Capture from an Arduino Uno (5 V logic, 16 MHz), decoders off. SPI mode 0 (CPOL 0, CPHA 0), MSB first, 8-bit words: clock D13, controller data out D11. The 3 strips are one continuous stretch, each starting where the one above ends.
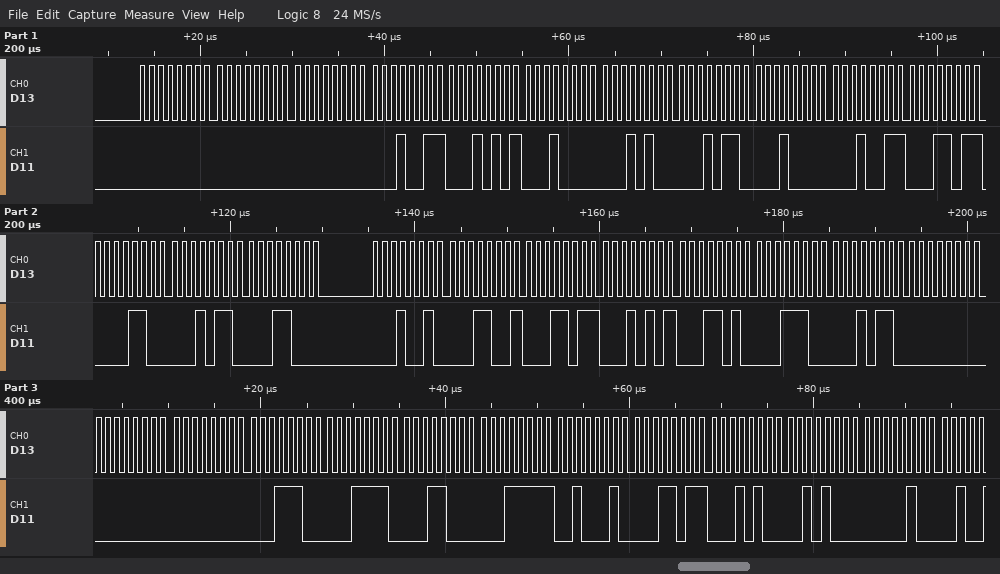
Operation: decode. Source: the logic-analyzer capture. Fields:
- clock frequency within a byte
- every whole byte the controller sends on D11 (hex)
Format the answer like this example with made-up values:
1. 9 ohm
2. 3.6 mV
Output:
1. 1 MHz
2. 0x00 0x00 0x00 0x13 0x15 0x10 0x14 0x16 0x10 0x13 0x1B 0x0C 0x16 0x18 0x12 0x19 0x1B 0x15 0x1A 0x1C 0x16 0x00 0x00 0x00 0x1C 0x1E 0x18 0x1F 0x22 0x1B 0x14 0x28 0x04
